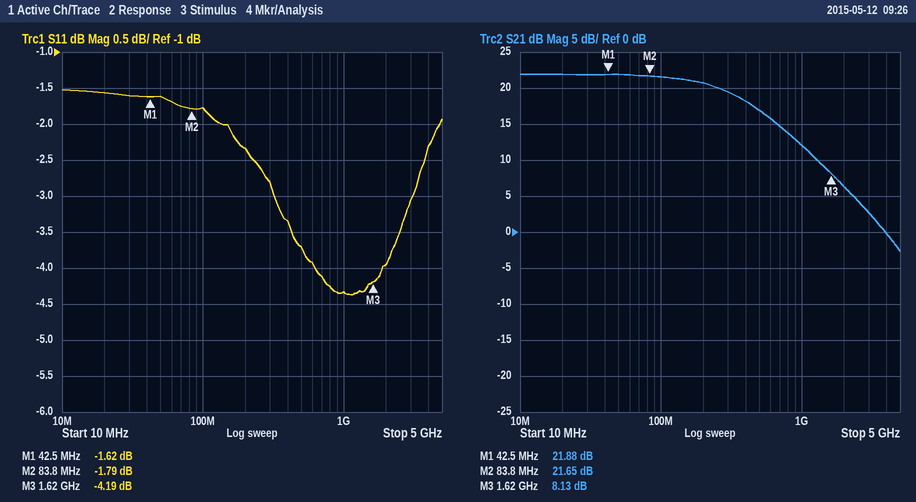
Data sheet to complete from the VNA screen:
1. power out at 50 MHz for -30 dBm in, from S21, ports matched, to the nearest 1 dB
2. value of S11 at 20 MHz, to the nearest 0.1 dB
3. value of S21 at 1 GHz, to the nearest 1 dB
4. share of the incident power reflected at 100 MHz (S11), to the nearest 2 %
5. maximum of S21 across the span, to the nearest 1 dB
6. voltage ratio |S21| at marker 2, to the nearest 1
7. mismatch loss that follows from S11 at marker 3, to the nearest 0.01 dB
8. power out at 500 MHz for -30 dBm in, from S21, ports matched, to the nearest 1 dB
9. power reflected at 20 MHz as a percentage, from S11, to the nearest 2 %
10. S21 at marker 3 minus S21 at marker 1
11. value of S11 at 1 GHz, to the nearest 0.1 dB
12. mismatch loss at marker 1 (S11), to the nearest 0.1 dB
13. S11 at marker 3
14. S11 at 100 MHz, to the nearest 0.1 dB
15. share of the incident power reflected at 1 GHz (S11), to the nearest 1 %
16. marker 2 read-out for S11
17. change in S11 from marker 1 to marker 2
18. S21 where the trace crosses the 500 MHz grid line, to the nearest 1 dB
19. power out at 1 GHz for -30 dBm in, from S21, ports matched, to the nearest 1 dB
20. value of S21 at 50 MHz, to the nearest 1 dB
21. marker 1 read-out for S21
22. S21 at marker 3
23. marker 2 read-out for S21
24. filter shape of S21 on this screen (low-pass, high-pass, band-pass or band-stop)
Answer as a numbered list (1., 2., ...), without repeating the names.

1. -8 dBm
2. -1.6 dB
3. 12 dB
4. 66 %
5. 22 dB
6. 12
7. 2.08 dB
8. -13 dBm
9. 70 %
10. -13.75 dB
11. -4.3 dB
12. 5.1 dB
13. -4.19 dB
14. -1.8 dB
15. 37 %
16. -1.79 dB
17. -0.17 dB
18. 17 dB
19. -18 dBm
20. 22 dB
21. 21.88 dB
22. 8.13 dB
23. 21.65 dB
24. low-pass
